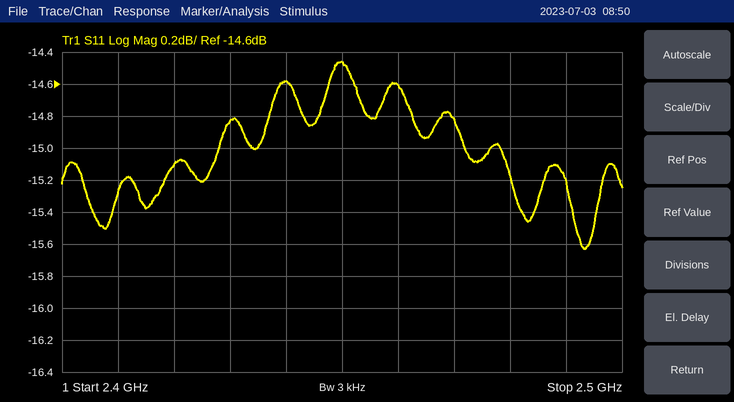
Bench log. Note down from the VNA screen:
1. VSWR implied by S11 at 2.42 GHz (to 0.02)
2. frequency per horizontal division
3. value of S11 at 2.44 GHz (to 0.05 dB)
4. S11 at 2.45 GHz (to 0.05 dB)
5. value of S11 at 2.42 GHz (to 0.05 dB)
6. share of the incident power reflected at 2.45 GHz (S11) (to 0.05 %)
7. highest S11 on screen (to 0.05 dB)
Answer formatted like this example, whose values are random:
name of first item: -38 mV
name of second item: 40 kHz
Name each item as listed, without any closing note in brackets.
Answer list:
VSWR implied by S11 at 2.42 GHz: 1.42
frequency per horizontal division: 10 MHz
value of S11 at 2.44 GHz: -14.60 dB
S11 at 2.45 GHz: -14.45 dB
value of S11 at 2.42 GHz: -15.10 dB
share of the incident power reflected at 2.45 GHz (S11): 3.60 %
highest S11 on screen: -14.45 dB
